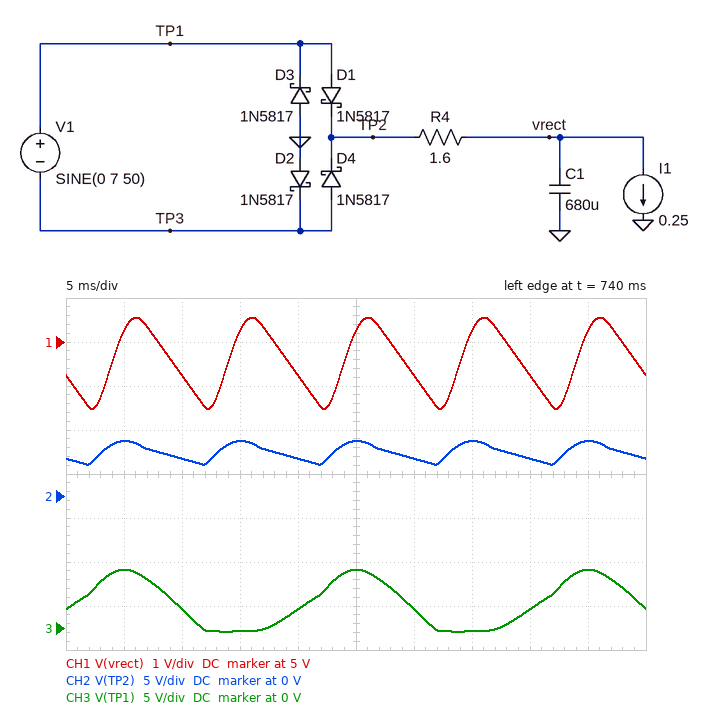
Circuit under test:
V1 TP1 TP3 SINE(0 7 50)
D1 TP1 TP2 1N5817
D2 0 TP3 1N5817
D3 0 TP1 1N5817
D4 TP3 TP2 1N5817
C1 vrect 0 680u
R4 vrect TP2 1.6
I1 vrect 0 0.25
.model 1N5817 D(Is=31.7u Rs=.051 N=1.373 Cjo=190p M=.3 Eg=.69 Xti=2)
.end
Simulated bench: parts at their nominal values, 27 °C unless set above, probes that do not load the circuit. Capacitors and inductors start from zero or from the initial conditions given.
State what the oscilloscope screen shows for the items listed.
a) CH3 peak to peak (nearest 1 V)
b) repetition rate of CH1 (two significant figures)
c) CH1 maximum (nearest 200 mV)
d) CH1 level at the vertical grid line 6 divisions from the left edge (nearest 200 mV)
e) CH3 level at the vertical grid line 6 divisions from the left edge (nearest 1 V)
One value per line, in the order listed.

7 V
100 Hz
5.6 V
4.2 V
2 V
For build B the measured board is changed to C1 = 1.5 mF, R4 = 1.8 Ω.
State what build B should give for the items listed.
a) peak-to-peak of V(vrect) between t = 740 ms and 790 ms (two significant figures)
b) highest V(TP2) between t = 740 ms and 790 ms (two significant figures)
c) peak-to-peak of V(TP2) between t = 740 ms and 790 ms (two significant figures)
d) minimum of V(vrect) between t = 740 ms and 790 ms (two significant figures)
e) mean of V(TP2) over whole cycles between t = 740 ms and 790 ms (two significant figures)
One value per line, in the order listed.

950 mV
6.2 V
2.0 V
4.2 V
5.1 V
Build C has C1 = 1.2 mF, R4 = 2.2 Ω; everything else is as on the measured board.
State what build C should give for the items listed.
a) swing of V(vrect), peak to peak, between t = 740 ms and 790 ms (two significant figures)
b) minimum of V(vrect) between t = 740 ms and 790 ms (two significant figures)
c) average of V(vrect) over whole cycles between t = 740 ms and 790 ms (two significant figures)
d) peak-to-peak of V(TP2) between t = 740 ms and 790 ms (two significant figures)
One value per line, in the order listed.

1.1 V
3.8 V
4.4 V
2.3 V
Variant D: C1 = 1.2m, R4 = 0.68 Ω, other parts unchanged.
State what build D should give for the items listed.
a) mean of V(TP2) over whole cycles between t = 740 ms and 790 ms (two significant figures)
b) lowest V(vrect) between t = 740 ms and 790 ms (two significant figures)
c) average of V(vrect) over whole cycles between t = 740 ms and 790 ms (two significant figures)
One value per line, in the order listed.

5.4 V
4.5 V
5.2 V
